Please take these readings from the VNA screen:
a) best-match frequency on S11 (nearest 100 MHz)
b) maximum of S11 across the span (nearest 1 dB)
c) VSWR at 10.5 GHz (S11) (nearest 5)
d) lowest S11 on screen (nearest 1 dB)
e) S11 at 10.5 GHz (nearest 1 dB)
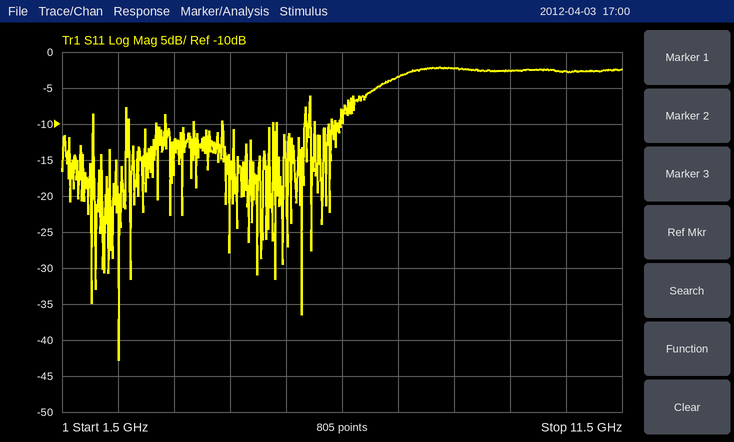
2.5 GHz
-2 dB
5
-43 dB
-3 dB
